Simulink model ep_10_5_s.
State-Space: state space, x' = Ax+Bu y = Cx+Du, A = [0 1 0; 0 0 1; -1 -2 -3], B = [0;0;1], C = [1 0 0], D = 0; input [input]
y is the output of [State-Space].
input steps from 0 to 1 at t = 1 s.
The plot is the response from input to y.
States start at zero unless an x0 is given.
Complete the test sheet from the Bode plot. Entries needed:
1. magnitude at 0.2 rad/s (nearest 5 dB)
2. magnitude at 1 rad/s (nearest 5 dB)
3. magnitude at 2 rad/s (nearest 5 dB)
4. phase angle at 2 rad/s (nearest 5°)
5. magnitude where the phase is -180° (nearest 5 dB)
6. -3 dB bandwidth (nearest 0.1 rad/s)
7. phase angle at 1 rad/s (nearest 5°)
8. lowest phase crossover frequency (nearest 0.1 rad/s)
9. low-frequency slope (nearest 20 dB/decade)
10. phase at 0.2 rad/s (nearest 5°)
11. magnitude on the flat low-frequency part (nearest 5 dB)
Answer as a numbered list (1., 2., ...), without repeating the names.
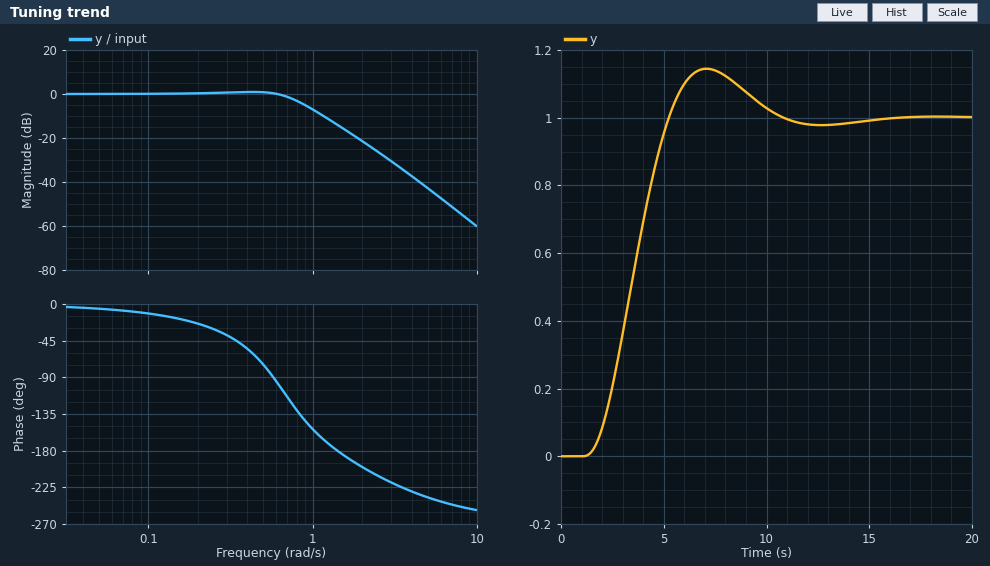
1. 0 dB
2. -5 dB
3. -20 dB
4. -200°
5. -15 dB
6. 0.8 rad/s
7. -155°
8. 1.4 rad/s
9. 0 dB/decade
10. -25°
11. 0 dB
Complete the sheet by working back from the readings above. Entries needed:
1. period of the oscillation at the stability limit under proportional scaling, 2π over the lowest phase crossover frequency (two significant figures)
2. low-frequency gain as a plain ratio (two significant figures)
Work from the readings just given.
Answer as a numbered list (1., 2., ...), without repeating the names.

1. 4.5 s
2. 1.0
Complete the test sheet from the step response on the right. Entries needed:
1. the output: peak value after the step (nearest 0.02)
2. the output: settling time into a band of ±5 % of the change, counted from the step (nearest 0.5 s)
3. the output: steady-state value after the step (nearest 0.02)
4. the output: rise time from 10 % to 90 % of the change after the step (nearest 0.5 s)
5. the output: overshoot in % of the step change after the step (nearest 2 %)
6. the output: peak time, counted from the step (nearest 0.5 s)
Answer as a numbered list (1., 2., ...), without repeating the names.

1. 1.14
2. 8.5 s
3. 1.00
4. 2.5 s
5. 14 %
6. 6.0 s
